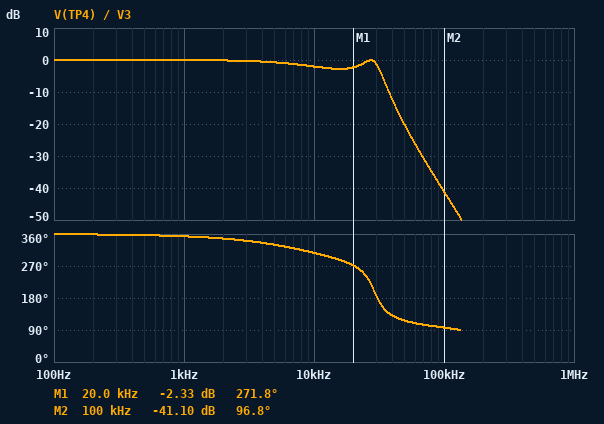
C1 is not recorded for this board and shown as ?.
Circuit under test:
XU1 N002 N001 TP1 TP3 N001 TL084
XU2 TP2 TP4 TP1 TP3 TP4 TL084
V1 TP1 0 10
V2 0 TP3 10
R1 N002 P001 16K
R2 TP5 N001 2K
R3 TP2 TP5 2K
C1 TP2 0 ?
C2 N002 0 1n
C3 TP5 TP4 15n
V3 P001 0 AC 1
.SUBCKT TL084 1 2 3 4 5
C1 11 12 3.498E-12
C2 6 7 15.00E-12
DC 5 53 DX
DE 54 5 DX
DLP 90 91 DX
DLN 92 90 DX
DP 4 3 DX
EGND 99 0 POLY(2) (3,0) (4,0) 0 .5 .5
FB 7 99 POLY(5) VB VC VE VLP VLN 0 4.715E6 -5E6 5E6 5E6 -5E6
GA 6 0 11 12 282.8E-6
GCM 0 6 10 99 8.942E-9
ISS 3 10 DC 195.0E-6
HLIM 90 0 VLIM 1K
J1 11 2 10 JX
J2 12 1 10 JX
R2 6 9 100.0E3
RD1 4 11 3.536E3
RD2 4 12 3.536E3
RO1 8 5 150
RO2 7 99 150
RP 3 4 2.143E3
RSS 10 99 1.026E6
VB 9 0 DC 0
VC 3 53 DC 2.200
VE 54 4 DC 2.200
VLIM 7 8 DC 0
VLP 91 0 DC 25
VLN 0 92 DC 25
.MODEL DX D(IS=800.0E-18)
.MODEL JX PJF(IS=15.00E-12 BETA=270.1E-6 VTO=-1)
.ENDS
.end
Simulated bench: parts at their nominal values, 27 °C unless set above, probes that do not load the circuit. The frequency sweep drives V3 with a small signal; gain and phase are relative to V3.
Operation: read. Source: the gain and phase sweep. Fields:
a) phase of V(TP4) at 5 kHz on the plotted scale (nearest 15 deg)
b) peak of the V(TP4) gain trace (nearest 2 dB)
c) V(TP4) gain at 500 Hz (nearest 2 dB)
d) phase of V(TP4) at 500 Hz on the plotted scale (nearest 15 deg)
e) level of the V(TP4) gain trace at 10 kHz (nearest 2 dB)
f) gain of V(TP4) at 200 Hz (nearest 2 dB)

330 deg
0 dB
0 dB
360 deg
-2 dB
0 dB
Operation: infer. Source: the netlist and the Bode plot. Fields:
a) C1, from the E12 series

470 pF
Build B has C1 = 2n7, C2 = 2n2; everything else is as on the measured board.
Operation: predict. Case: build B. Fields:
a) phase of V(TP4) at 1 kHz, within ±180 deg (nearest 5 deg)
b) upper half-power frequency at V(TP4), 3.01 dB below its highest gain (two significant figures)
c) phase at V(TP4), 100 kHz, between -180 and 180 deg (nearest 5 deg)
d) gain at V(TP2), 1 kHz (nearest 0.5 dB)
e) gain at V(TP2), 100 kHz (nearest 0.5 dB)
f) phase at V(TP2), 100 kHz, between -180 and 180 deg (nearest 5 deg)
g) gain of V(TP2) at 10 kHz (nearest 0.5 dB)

-15 deg
5.7 kHz
85 deg
0 dB
-63.5 dB
95 deg
-5.5 dB
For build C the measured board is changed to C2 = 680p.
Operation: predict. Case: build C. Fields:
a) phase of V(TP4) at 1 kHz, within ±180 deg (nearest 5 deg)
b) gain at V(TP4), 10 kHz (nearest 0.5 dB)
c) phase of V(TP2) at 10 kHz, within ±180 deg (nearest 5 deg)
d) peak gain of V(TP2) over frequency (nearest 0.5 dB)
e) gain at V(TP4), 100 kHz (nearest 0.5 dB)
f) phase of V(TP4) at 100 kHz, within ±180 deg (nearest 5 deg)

-5 deg
-0.5 dB
-40 deg
2.5 dB
-38.0 dB
100 deg
